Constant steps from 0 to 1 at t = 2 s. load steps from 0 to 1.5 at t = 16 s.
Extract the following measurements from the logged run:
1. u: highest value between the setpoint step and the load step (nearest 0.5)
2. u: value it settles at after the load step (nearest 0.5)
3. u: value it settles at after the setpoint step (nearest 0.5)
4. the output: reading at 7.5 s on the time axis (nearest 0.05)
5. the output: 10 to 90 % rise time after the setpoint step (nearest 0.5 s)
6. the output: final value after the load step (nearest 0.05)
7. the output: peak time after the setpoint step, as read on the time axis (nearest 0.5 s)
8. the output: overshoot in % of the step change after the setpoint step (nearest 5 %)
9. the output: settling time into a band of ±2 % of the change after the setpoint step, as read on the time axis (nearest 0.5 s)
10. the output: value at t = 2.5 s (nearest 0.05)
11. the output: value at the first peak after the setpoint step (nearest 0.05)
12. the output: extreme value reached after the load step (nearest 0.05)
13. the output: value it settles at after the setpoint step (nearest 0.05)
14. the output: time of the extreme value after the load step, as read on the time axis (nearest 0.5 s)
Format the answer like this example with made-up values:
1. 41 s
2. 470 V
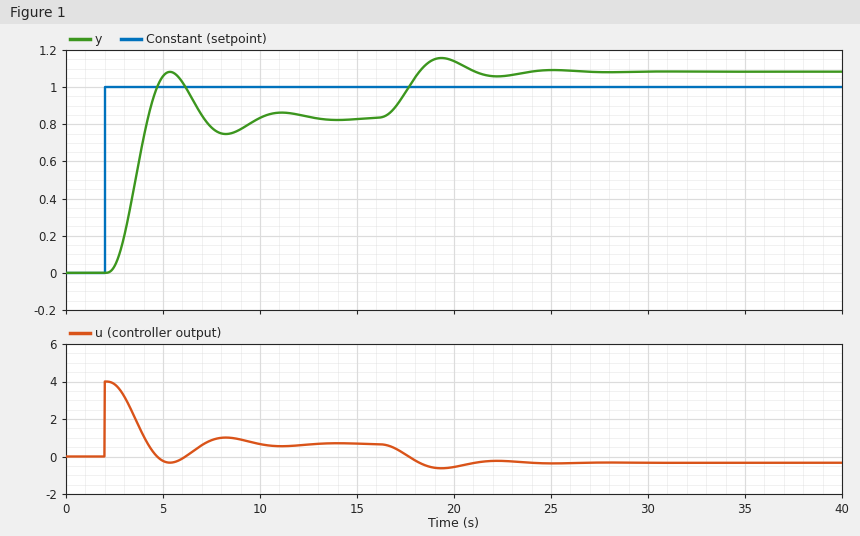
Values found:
1. 4.0
2. -0.5
3. 0.5
4. 0.80
5. 1.5 s
6. 1.10
7. 5.5 s
8. 30 %
9. 12.0 s
10. 0.05
11. 1.10
12. 1.15
13. 0.85
14. 19.5 s
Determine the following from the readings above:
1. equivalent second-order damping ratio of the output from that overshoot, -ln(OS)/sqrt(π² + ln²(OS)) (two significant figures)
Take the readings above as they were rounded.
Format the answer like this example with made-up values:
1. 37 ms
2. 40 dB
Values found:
1. 0.36
